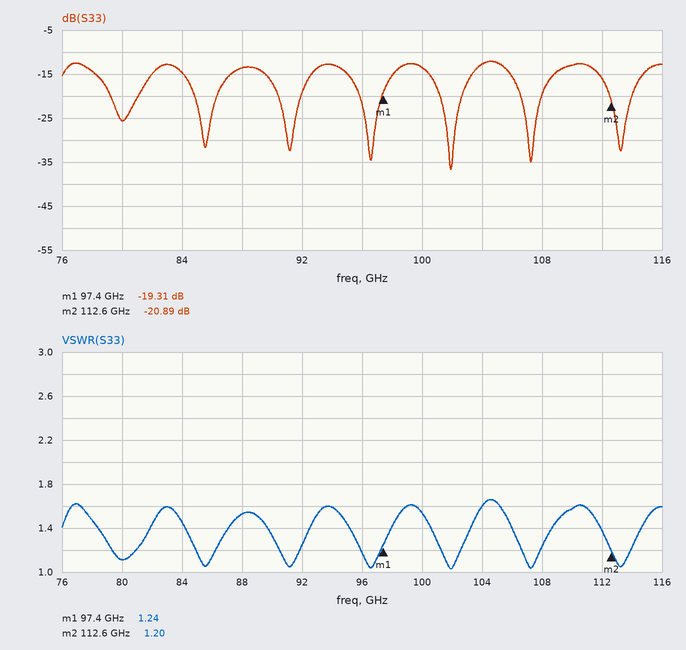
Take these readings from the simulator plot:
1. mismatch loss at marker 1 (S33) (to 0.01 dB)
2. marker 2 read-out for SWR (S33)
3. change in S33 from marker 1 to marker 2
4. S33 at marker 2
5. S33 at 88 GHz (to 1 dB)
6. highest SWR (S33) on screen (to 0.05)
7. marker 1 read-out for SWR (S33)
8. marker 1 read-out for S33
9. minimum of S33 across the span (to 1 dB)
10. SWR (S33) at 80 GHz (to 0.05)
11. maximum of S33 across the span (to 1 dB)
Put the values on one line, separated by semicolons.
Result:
0.05 dB; 1.20; -1.58 dB; -20.89 dB; -14 dB; 1.65; 1.24; -19.31 dB; -37 dB; 1.10; -12 dB
